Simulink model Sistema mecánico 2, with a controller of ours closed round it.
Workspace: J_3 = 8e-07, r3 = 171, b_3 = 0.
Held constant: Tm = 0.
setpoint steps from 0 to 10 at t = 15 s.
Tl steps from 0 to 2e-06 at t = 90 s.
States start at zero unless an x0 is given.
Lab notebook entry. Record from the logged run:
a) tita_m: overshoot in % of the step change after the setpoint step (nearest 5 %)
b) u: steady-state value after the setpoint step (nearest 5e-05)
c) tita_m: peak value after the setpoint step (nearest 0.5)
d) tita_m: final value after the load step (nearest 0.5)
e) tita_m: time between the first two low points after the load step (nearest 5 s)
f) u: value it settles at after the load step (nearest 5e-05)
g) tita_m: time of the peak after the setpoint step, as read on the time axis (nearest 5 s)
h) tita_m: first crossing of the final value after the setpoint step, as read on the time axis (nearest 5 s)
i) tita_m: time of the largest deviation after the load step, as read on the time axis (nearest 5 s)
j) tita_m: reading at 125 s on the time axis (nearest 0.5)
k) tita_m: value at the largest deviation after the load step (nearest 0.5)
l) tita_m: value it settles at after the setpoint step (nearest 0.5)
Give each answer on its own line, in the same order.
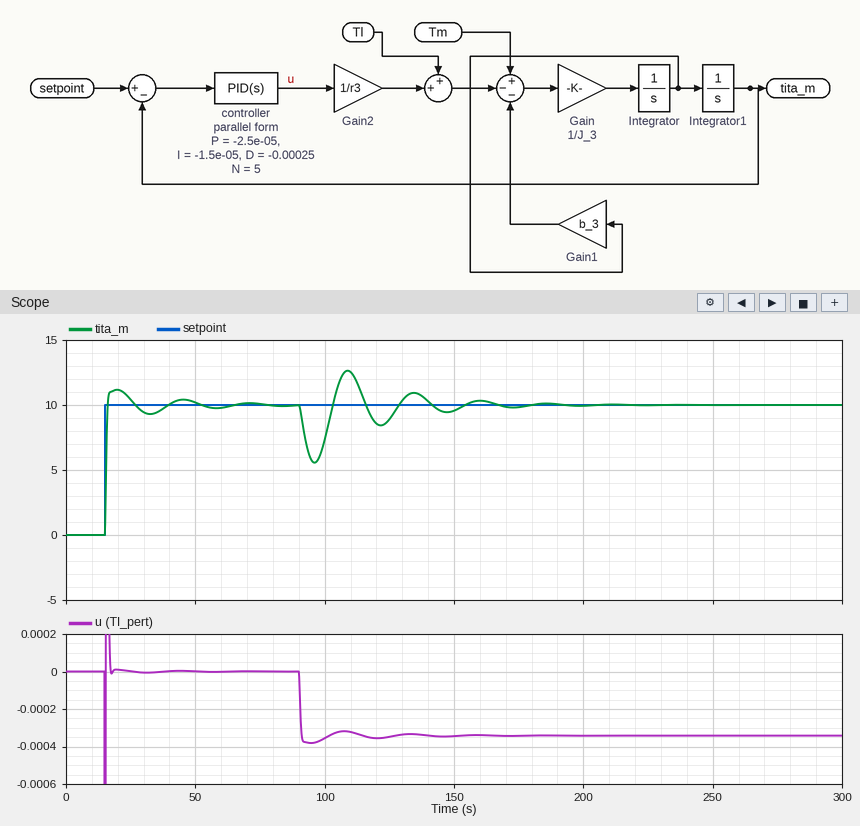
10 %
0.00000
11.0
10.0
25 s
-0.00035
20 s
15 s
95 s
9.0
5.5
10.0
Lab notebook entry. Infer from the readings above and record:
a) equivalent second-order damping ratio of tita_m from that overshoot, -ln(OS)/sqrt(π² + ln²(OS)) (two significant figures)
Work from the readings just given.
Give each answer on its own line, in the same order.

0.59
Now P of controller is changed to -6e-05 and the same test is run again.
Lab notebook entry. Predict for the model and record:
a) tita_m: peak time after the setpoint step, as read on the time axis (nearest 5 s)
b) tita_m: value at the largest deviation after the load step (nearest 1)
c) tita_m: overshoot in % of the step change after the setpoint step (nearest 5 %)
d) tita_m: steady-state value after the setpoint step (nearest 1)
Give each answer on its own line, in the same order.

15 s
7
15 %
10
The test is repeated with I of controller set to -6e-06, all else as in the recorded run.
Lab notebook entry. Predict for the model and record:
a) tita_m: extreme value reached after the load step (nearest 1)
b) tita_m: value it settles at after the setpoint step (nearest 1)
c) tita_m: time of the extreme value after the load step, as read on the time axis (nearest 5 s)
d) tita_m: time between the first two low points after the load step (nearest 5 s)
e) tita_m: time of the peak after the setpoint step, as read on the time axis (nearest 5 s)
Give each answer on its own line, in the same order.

4
10
100 s
40 s
15 s
